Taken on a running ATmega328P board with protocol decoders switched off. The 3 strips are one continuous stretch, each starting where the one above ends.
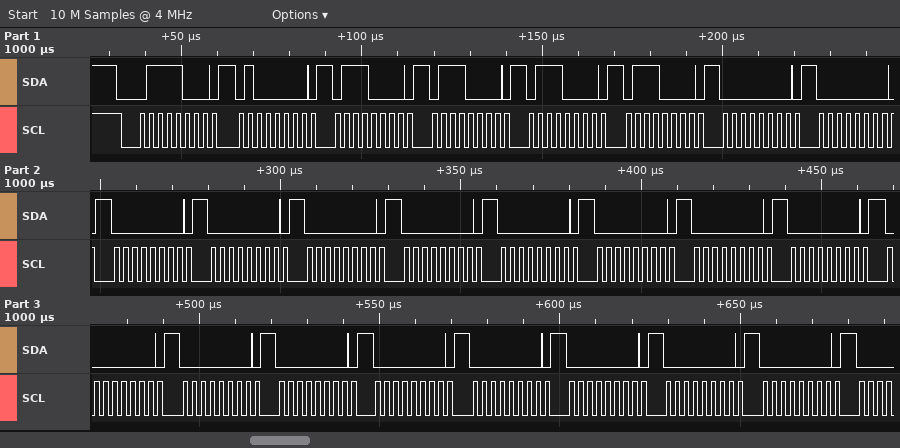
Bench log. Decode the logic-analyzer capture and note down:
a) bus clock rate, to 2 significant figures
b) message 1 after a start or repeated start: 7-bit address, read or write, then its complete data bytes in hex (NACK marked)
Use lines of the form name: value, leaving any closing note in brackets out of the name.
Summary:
bus clock rate, to 2 significant figures: 400 kHz
message 1 after a start or repeated start: 7-bit address, read or write, then its complete data bytes in hex: 0x3C write: 40 70 70 70 70 00 00 00 00 00 00 00 00 00 00 00 00 00 00 00 00 00 00
